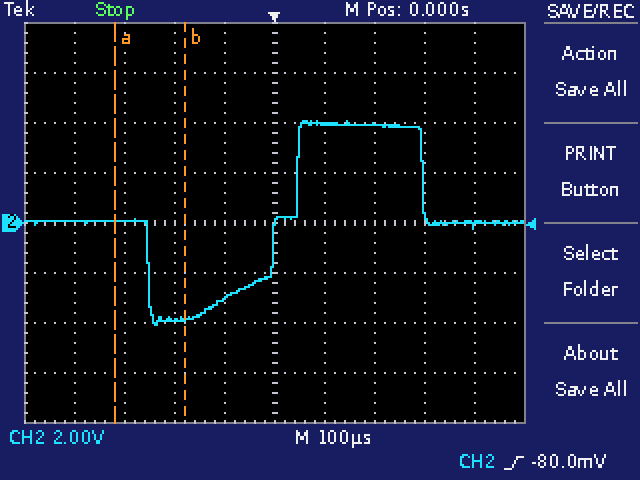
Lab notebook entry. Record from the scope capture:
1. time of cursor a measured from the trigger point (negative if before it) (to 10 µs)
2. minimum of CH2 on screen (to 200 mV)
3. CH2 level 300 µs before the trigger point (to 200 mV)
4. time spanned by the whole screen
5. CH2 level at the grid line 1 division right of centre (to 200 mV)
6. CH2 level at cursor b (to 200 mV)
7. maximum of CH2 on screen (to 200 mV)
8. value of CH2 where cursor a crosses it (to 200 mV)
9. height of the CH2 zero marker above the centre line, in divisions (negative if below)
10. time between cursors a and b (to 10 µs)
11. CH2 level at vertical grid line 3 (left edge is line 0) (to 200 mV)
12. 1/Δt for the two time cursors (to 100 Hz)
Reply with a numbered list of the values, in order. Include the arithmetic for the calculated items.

1. -320 µs
2. -4.0 V
3. 0.0 V
4. 1 ms
5. 4.0 V
6. -3.8 V
7. 4.0 V
8. 0.0 V
9. 0.0 div
10. 140 µs
11. -3.8 V
12. 1 / 140 µs ≈ 7.1 kHz
